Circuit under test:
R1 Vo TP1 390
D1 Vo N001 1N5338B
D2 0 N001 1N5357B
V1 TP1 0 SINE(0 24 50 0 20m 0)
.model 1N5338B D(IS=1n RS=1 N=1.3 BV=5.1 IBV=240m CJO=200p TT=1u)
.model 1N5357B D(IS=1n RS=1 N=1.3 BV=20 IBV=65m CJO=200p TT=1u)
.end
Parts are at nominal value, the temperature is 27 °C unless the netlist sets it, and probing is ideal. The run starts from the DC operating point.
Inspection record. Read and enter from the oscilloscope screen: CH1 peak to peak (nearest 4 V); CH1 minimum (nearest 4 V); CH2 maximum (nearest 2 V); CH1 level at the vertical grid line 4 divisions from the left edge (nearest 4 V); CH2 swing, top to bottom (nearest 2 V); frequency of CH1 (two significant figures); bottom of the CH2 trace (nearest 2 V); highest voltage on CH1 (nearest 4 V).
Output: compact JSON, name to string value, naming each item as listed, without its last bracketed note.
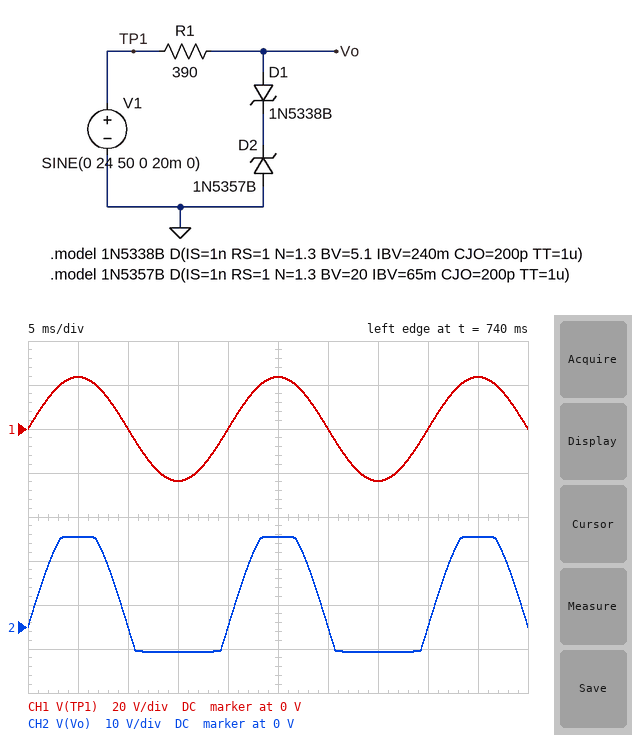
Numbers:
{"CH1 peak to peak": "48 V", "CH1 minimum": "-24 V", "CH2 maximum": "20 V", "CH1 level at the vertical grid line 4 divisions from the left edge": "0 V", "CH2 swing, top to bottom": "26 V", "frequency of CH1": "50 Hz", "bottom of the CH2 trace": "-6 V", "highest voltage on CH1": "24 V"}
